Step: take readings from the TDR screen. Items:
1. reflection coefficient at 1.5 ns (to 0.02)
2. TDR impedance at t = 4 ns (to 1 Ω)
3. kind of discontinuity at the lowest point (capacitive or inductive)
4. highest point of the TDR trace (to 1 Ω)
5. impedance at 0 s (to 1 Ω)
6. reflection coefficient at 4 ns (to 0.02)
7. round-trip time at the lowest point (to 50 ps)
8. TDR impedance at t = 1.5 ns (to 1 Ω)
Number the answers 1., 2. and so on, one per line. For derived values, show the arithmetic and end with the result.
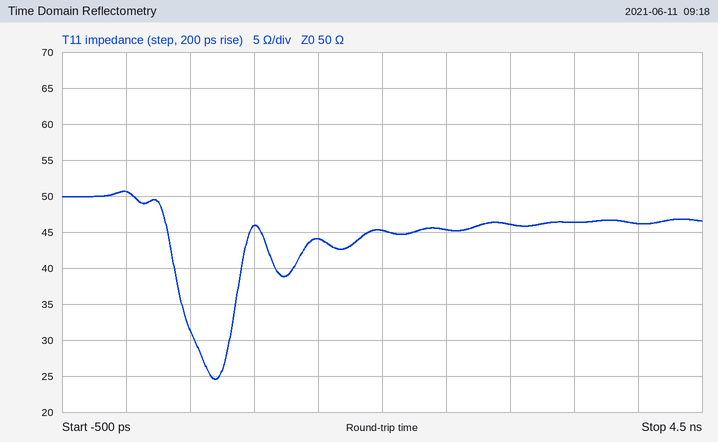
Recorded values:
1. (44 − 50)/(44 + 50) ≈ -0.06
2. 46 Ω
3. capacitive
4. 51 Ω
5. 51 Ω
6. (46 − 50)/(46 + 50) ≈ -0.04
7. 700 ps
8. 44 Ω
